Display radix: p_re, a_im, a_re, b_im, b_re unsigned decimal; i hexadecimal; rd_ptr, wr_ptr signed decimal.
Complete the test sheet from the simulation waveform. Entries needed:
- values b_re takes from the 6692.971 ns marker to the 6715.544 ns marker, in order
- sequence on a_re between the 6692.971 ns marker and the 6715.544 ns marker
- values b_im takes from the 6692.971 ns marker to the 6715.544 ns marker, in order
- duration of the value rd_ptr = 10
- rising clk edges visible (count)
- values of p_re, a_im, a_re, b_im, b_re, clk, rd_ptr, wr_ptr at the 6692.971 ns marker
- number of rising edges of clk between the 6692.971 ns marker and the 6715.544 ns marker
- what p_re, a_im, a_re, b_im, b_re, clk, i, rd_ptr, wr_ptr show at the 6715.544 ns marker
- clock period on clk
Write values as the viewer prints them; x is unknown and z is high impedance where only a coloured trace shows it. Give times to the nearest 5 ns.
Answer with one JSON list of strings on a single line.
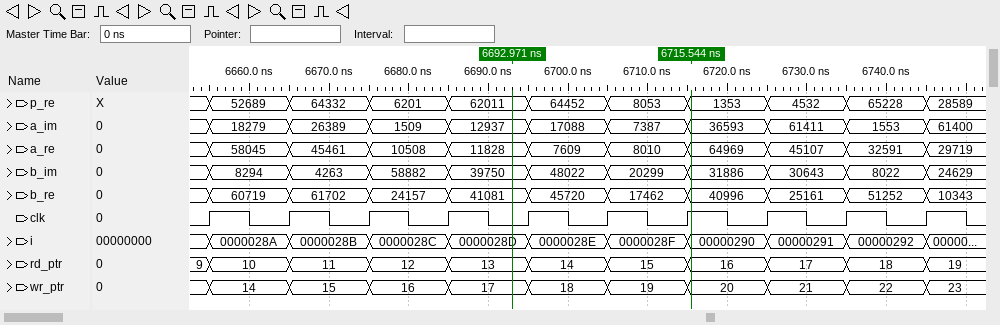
["41081, 45720, 17462, 40996", "11828, 7609, 8010, 64969", "39750, 48022, 20299, 31886", "10 ns", "10", "p_re=62011, a_im=12937, a_re=11828, b_im=39750, b_re=41081, clk=0, rd_ptr=13, wr_ptr=17", "3", "p_re=1353, a_im=36593, a_re=64969, b_im=31886, b_re=40996, clk=1, i=00000290, rd_ptr=16, wr_ptr=20", "10 ns"]
